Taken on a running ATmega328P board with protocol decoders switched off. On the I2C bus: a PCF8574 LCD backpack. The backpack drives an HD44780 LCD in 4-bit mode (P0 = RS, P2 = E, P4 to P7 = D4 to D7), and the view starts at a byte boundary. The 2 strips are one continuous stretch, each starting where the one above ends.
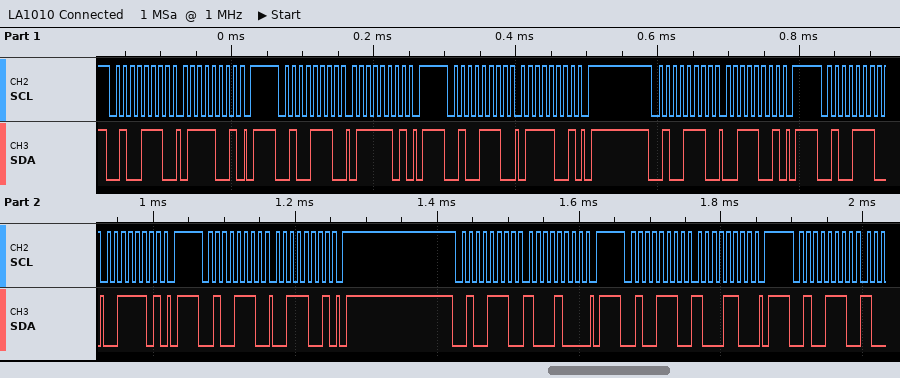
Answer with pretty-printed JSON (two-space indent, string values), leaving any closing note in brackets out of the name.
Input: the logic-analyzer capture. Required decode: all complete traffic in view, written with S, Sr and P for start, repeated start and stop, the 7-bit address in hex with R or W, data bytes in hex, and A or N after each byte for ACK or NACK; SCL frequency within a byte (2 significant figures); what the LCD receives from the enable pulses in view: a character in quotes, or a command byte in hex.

{
  "all complete traffic in view, written with S, Sr and P for start, repeated start and stop, the 7-bit address in hex with R or W, data bytes in hex, and A or N after each byte for ACK or NACK": "S 27W A 79 A P S 27W A 7D A P S 27W A 79 A P S 27W A 39 A P S 27W A 3D A P S 27W A 39 A P S 27W A 88 A P S 27W A 8C A P S 27W A",
  "SCL frequency within a byte": "100 kHz",
  "what the LCD receives from the enable pulses in view: a character in quotes, or a command byte in hex": "'s'"
}
